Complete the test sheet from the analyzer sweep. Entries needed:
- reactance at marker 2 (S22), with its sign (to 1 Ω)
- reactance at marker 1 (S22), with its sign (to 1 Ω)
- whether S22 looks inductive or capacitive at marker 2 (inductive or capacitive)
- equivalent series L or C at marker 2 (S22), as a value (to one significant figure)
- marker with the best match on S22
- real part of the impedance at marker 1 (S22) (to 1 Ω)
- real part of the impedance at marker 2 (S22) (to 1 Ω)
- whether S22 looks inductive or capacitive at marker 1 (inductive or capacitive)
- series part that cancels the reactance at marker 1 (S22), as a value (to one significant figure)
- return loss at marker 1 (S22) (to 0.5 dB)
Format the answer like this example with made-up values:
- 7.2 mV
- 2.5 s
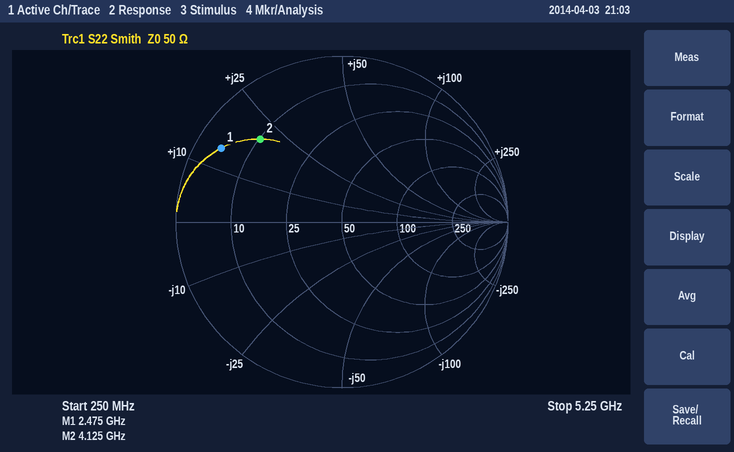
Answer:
- +20 Ω
- +14 Ω
- inductive
- 800 pH
- marker 2
- 4 Ω
- 10 Ω
- inductive
- 5 pF
- 1.5 dB
